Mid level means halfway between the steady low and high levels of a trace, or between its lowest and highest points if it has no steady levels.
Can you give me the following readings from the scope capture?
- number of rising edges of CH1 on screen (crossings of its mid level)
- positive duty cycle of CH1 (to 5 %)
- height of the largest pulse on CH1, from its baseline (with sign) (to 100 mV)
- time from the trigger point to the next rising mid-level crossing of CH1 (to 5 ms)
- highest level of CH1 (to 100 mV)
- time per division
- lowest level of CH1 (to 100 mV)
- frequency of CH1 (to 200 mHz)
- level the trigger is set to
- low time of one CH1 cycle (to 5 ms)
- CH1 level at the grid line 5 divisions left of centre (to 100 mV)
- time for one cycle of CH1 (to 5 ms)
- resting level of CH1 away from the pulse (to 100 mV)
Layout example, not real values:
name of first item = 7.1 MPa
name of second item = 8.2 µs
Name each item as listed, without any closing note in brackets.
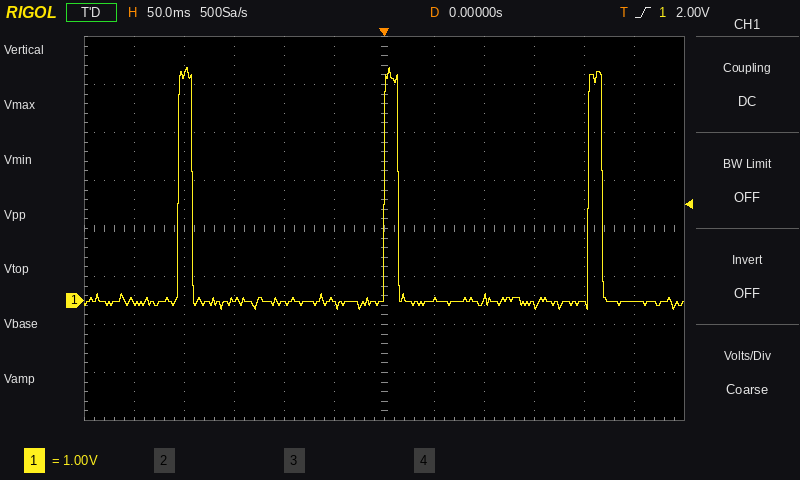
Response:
number of rising edges of CH1 on screen = 3
positive duty cycle of CH1 = 5 %
height of the largest pulse on CH1, from its baseline (with sign) = +4.9 V
time from the trigger point to the next rising mid-level crossing of CH1 = 205 ms
highest level of CH1 = 4.9 V
time per division = 50 ms
lowest level of CH1 = -200 mV
frequency of CH1 = 4.8 Hz
level the trigger is set to = 2.00 V
low time of one CH1 cycle = 190 ms
CH1 level at the grid line 5 divisions left of centre = 0.0 V
time for one cycle of CH1 = 205 ms
resting level of CH1 away from the pulse = 0.0 V
